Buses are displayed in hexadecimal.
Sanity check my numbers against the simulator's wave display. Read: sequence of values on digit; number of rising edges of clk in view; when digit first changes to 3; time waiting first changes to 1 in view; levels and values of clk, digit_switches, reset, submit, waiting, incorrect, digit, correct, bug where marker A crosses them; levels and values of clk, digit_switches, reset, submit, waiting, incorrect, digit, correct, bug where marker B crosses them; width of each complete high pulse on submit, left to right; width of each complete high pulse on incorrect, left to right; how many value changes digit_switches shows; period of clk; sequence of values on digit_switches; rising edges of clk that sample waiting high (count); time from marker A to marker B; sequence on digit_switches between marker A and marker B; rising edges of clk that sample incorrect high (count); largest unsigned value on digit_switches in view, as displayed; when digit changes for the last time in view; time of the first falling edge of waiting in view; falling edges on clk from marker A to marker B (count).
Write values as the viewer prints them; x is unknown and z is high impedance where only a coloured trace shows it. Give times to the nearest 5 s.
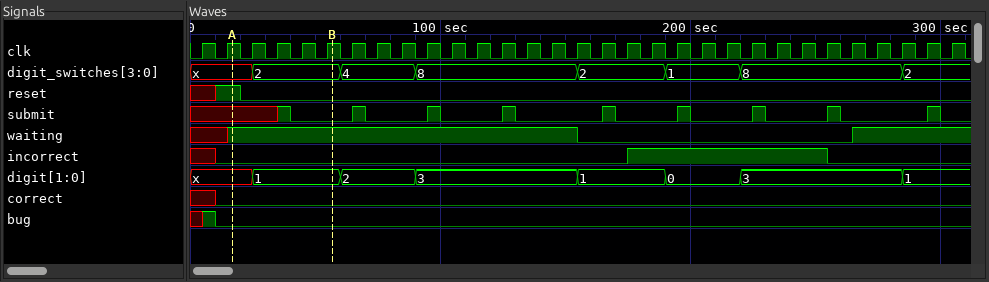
x, 1, 2, 3, 1, 0, 3, 1
31
90 s
15 s
clk=1, digit_switches=x, reset=1, submit=x, waiting=1, incorrect=0, digit=x, correct=0, bug=0
clk=1, digit_switches=2, reset=0, submit=0, waiting=1, incorrect=0, digit=1, correct=0, bug=0
5 s, 5 s, 5 s, 5 s, 5 s, 5 s, 5 s, 5 s
80 s
7
10 s
x, 2, 4, 8, 2, 1, 8, 2
18
40 s
x, 2
8
8
285 s
155 s
4
